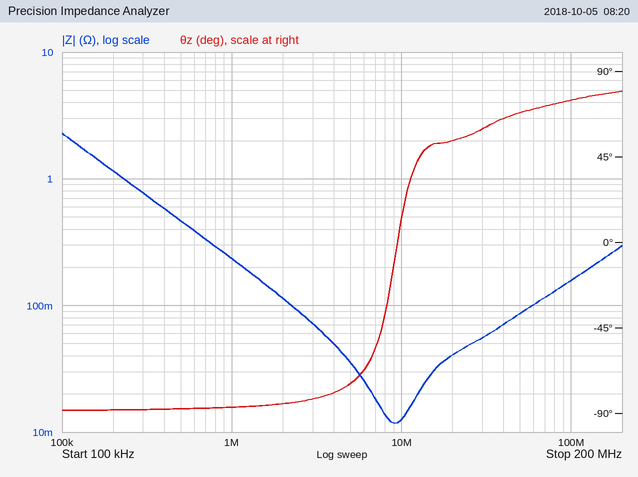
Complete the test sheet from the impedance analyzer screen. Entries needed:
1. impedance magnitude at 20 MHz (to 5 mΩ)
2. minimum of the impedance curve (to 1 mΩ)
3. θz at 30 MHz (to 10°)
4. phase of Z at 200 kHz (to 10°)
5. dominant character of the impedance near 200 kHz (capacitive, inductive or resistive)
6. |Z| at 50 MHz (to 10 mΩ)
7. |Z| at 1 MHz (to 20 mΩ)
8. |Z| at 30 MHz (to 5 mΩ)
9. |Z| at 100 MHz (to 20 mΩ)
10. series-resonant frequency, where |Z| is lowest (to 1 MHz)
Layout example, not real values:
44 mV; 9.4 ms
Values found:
40 mΩ; 12 mΩ; 60°; -90°; capacitive; 90 mΩ; 240 mΩ; 55 mΩ; 160 mΩ; 9 MHz
